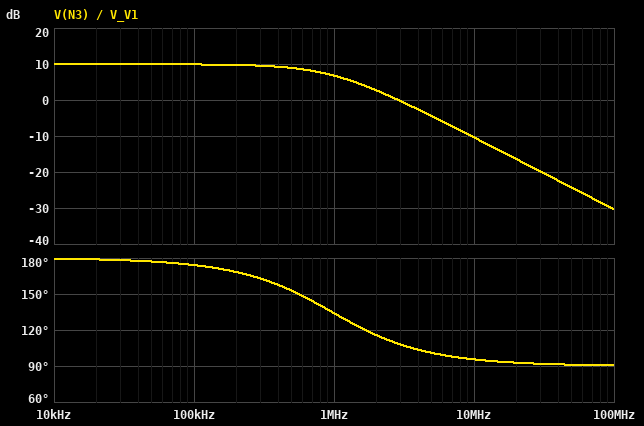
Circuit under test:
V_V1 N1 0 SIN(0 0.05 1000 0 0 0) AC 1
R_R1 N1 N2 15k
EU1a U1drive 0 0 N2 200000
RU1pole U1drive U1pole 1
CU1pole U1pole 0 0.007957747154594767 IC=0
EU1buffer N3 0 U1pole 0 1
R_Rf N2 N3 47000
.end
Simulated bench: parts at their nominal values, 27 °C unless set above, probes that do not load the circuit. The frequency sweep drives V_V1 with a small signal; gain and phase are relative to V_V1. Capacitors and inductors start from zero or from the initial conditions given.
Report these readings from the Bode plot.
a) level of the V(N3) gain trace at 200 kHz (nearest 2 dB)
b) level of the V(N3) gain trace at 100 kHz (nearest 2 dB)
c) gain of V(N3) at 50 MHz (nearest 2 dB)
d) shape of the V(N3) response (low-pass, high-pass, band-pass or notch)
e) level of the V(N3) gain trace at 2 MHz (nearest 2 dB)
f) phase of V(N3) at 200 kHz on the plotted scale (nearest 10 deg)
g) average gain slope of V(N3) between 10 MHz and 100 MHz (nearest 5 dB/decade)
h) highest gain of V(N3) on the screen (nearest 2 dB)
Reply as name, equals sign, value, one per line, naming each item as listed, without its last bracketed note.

level of the V(N3) gain trace at 200 kHz = 10 dB
level of the V(N3) gain trace at 100 kHz = 10 dB
gain of V(N3) at 50 MHz = -24 dB
shape of the V(N3) response = low-pass
level of the V(N3) gain trace at 2 MHz = 2 dB
phase of V(N3) at 200 kHz on the plotted scale = 170 deg
average gain slope of V(N3) between 10 MHz and 100 MHz = -20 dB/decade
highest gain of V(N3) on the screen = 10 dB
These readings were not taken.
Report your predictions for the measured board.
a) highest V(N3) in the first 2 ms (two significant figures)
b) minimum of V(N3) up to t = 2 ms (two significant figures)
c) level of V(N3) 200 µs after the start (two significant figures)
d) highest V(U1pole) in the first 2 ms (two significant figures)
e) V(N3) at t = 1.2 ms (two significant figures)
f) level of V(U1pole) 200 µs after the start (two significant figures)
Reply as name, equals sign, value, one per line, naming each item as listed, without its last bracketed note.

highest V(N3) in the first 2 ms = 160 mV
minimum of V(N3) up to t = 2 ms = -160 mV
level of V(N3) 200 µs after the start = -150 mV
highest V(U1pole) in the first 2 ms = 160 mV
V(N3) at t = 1.2 ms = -150 mV
level of V(U1pole) 200 µs after the start = -150 mV
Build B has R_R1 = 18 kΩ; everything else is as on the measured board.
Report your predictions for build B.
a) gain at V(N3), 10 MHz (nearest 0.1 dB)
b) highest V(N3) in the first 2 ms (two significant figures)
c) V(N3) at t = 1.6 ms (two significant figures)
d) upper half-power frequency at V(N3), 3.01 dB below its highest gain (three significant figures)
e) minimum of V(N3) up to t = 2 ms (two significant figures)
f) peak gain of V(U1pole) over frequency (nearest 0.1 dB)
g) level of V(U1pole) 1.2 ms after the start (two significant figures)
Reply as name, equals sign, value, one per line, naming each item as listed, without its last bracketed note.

gain at V(N3), 10 MHz = -10.8 dB
highest V(N3) in the first 2 ms = 130 mV
V(N3) at t = 1.6 ms = 77 mV
upper half-power frequency at V(N3), 3.01 dB below its highest gain = 1.11 MHz
minimum of V(N3) up to t = 2 ms = -130 mV
peak gain of V(U1pole) over frequency = 8.3 dB
level of V(U1pole) 1.2 ms after the start = -120 mV
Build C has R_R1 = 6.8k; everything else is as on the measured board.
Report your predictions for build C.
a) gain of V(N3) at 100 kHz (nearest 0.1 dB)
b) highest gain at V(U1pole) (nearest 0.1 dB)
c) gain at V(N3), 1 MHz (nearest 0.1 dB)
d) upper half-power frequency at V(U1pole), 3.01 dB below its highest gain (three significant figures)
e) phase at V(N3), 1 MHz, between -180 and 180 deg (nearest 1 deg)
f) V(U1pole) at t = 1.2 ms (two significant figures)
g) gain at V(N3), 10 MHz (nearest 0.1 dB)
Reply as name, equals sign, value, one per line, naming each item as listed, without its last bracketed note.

gain of V(N3) at 100 kHz = 16.6 dB
highest gain at V(U1pole) = 16.8 dB
gain at V(N3), 1 MHz = 9.9 dB
upper half-power frequency at V(U1pole), 3.01 dB below its highest gain = 506 kHz
phase at V(N3), 1 MHz, between -180 and 180 deg = 117 deg
V(U1pole) at t = 1.2 ms = -330 mV
gain at V(N3), 10 MHz = -9.1 dB
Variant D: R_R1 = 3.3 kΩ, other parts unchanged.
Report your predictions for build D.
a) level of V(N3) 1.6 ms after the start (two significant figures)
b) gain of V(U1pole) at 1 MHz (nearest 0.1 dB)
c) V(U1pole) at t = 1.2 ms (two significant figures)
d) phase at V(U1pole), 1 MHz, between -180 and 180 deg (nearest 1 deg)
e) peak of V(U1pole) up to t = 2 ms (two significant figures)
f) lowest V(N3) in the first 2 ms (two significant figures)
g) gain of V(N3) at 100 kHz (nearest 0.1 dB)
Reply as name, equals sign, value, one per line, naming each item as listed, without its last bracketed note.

level of V(N3) 1.6 ms after the start = 420 mV
gain of V(U1pole) at 1 MHz = 11.2 dB
V(U1pole) at t = 1.2 ms = -680 mV
phase at V(U1pole), 1 MHz, between -180 and 180 deg = 105 deg
peak of V(U1pole) up to t = 2 ms = 710 mV
lowest V(N3) in the first 2 ms = -710 mV
gain of V(N3) at 100 kHz = 22.5 dB
